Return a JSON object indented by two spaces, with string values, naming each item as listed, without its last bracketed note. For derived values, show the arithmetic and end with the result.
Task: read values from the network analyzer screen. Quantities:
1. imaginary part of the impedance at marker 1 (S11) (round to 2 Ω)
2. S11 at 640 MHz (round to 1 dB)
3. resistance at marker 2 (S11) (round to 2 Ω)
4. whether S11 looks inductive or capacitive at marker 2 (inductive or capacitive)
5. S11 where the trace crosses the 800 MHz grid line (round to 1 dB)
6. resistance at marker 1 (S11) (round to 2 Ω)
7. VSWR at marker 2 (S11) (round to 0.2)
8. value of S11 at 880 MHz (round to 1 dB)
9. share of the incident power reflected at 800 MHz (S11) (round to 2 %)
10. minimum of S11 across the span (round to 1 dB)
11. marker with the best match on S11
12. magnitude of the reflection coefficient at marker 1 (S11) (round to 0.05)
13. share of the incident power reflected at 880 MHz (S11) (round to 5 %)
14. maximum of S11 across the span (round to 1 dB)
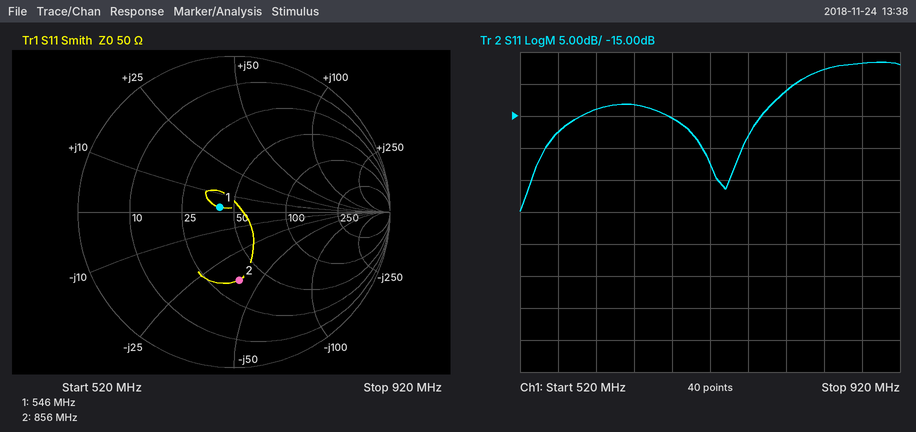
{
  "imaginary part of the impedance at marker 1 (S11)": "+2 Ω",
  "S11 at 640 MHz": "-13 dB",
  "resistance at marker 2 (S11)": "36 Ω",
  "whether S11 looks inductive or capacitive at marker 2": "capacitive",
  "S11 where the trace crosses the 800 MHz grid line": "-11 dB",
  "resistance at marker 1 (S11)": "42 Ω",
  "VSWR at marker 2 (S11)": "2.6",
  "value of S11 at 880 MHz": "-7 dB",
  "share of the incident power reflected at 800 MHz (S11)": "10^(-11/10) ≈ 8 %",
  "minimum of S11 across the span": "-30 dB",
  "marker with the best match on S11": "marker 1",
  "magnitude of the reflection coefficient at marker 1 (S11)": "0.10",
  "share of the incident power reflected at 880 MHz (S11)": "10^(-7/10) ≈ 20 %",
  "maximum of S11 across the span": "-7 dB"
}
